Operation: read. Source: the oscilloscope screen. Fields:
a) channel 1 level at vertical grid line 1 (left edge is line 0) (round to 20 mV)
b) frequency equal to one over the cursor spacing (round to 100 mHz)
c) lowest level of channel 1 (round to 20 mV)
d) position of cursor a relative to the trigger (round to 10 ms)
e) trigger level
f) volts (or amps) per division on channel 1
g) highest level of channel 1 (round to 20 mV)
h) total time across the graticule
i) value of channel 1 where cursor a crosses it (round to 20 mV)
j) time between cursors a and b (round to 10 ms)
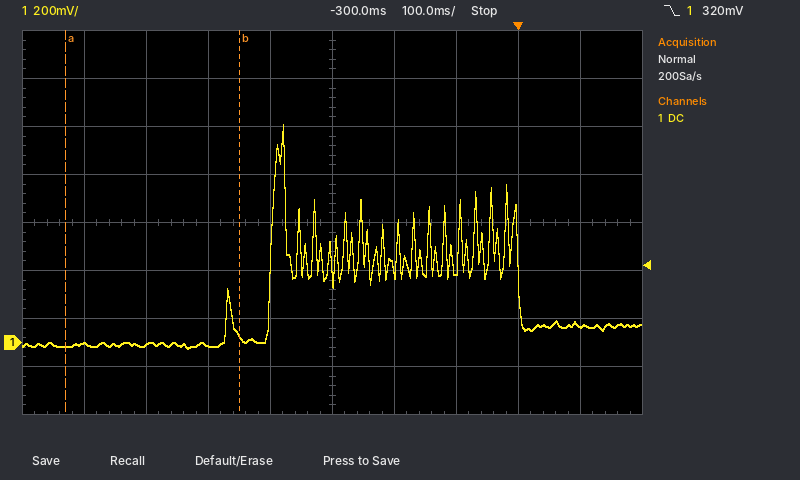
0 mV
3.6 Hz
-20 mV
-730 ms
320 mV
200 mV
900 mV
1 s
-20 mV
280 ms
